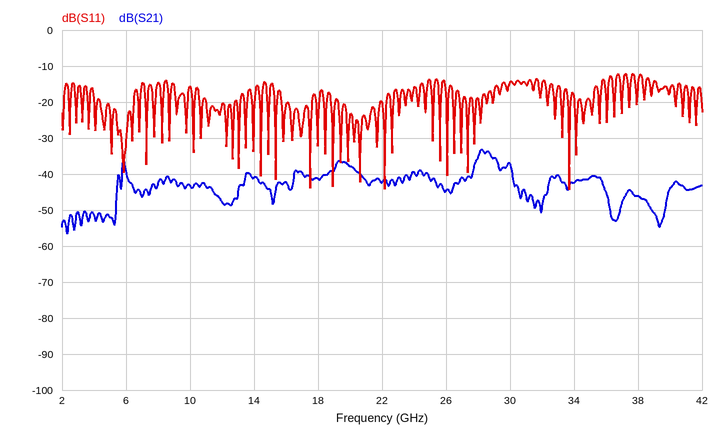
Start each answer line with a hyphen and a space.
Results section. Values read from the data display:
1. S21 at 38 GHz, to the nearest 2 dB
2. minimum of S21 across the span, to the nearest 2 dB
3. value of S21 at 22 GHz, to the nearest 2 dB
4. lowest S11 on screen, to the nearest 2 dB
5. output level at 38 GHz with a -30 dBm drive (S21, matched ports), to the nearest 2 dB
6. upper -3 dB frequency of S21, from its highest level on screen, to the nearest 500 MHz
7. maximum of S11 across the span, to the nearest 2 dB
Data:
- -46 dB
- -56 dB
- -42 dB
- -44 dB
- -76 dBm
- 29.0 GHz
- -12 dB
